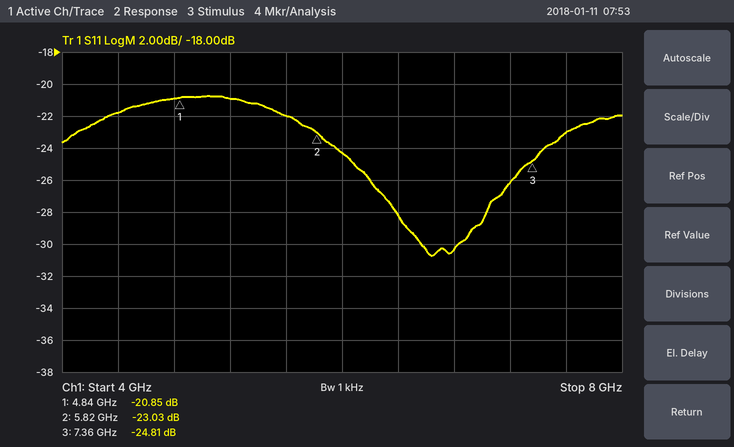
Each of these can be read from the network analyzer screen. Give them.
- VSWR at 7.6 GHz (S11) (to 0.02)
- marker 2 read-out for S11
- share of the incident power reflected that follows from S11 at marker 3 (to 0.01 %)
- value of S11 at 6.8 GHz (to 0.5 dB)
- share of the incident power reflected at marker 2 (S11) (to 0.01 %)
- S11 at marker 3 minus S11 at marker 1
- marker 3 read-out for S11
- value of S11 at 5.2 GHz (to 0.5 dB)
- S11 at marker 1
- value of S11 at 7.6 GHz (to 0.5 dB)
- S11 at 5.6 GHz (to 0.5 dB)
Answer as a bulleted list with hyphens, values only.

- 1.16
- -23.03 dB
- 0.33 %
- -30.5 dB
- 0.50 %
- -3.96 dB
- -24.81 dB
- -21.0 dB
- -20.85 dB
- -23.0 dB
- -22.0 dB
